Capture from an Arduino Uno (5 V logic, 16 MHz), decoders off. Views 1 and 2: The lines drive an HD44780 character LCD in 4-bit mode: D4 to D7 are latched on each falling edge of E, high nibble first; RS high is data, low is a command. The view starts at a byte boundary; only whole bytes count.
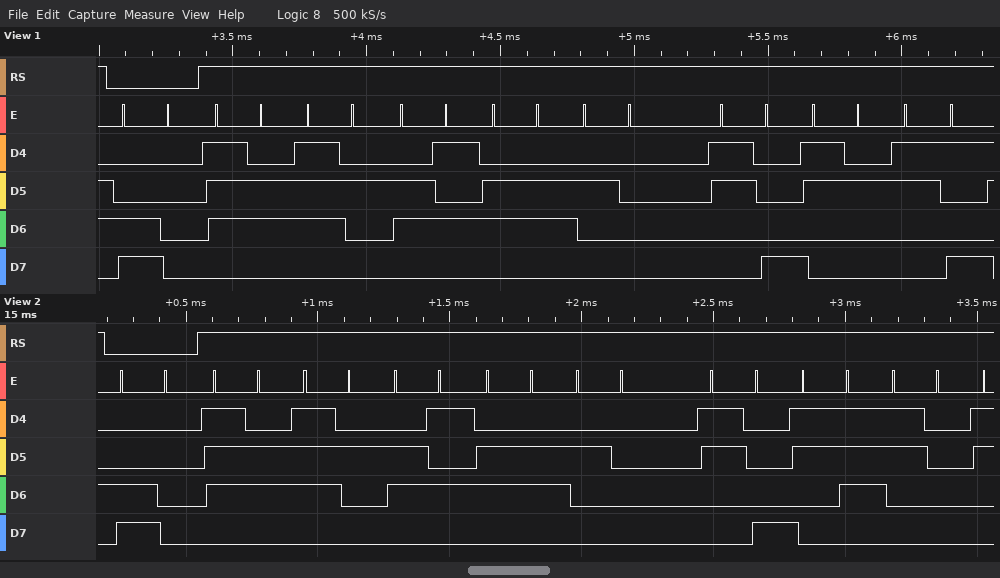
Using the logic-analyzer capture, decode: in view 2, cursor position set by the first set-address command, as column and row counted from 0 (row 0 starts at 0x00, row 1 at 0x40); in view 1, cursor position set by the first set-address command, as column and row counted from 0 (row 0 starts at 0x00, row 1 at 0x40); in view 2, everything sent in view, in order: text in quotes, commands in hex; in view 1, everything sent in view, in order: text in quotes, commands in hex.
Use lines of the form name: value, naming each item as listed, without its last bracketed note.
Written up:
in view 2, cursor position set by the first set-address command, as column and row counted from 0: column 0, row 1
in view 1, cursor position set by the first set-address command, as column and row counted from 0: column 0, row 1
in view 2, everything sent in view, in order: text in quotes, commands in hex: 0xC0 "vref 870"
in view 1, everything sent in view, in order: text in quotes, commands in hex: 0xC0 "vref 829"
